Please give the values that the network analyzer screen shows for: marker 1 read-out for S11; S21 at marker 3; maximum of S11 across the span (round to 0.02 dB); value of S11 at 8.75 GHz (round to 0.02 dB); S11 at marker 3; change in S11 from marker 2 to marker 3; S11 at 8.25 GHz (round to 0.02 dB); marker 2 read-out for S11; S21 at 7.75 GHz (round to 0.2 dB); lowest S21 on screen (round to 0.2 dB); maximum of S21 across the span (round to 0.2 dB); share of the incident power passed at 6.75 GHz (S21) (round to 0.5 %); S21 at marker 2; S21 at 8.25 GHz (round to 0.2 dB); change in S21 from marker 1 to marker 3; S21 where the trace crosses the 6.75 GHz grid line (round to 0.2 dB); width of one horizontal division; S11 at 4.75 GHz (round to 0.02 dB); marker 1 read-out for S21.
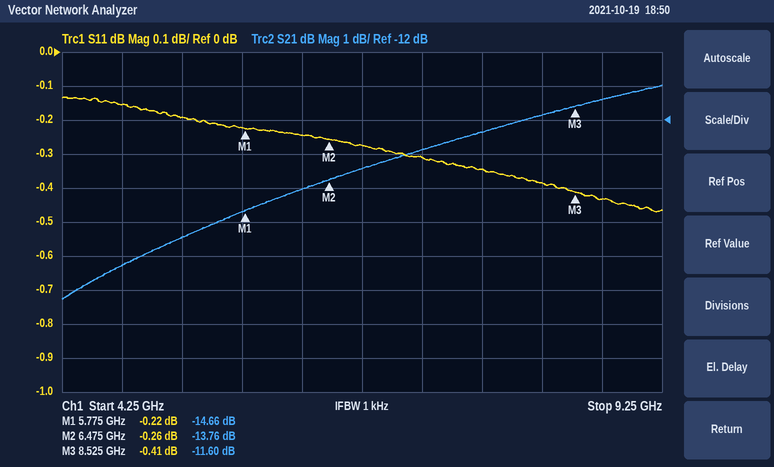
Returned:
-0.22 dB
-11.60 dB
-0.14 dB
-0.44 dB
-0.41 dB
-0.15 dB
-0.38 dB
-0.26 dB
-12.4 dB
-17.2 dB
-11.0 dB
4.5 %
-13.76 dB
-11.8 dB
3.06 dB
-13.4 dB
500 MHz
-0.16 dB
-14.66 dB
